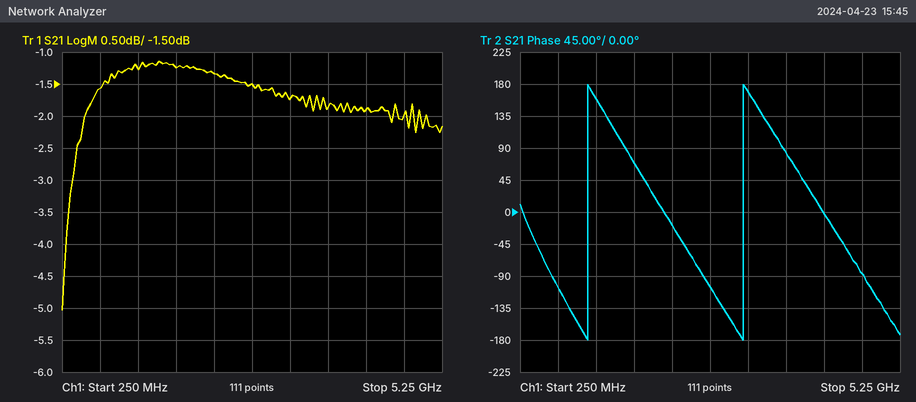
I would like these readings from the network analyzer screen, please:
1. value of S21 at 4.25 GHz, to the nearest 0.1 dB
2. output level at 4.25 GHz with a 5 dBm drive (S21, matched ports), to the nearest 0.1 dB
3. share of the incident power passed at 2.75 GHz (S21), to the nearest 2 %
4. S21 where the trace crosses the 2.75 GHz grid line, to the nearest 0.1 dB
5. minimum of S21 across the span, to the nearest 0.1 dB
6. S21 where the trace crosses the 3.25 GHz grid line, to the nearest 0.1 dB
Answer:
-1.9 dB
3.1 dBm
70 %
-1.5 dB
-5.0 dB
-1.7 dB
